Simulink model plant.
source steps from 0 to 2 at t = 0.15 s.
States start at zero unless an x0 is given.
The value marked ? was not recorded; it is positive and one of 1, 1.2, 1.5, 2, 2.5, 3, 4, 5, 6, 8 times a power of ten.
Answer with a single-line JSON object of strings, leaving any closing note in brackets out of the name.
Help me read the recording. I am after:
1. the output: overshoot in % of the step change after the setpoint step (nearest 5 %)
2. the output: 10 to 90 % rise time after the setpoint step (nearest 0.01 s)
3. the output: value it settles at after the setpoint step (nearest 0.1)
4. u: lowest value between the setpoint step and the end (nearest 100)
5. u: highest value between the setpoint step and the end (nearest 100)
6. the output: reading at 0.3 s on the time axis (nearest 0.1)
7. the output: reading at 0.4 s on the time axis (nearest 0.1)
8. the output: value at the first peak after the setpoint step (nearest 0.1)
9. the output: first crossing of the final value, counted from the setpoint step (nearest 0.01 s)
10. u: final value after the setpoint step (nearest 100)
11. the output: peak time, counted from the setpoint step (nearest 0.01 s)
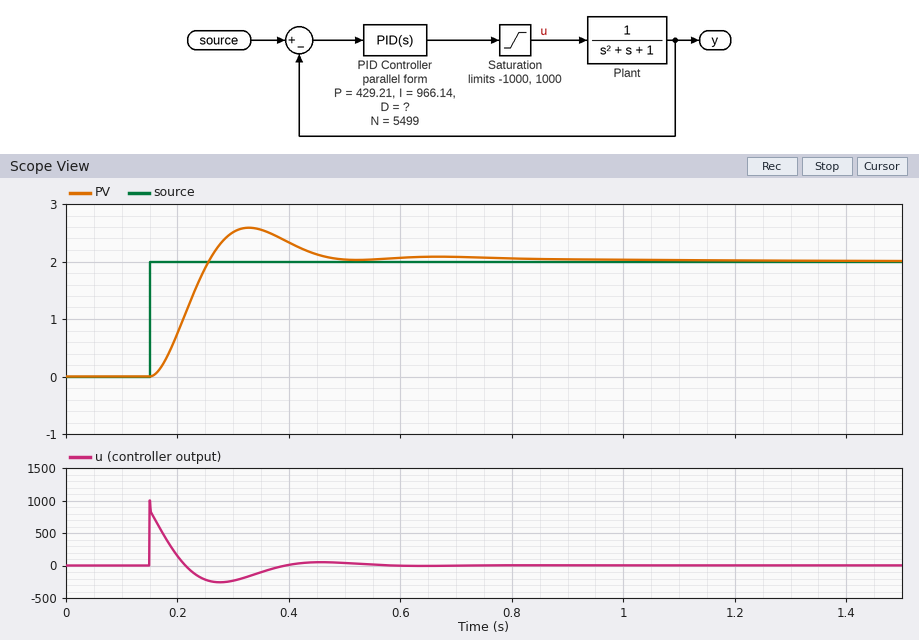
{"the output: overshoot in % of the step change after the setpoint step": "30 %", "the output: 10 to 90 % rise time after the setpoint step": "0.07 s", "the output: value it settles at after the setpoint step": "2.0", "u: lowest value between the setpoint step and the end": "-300", "u: highest value between the setpoint step and the end": "1000", "the output: reading at 0.3 s on the time axis": "2.5", "the output: reading at 0.4 s on the time axis": "2.3", "the output: value at the first peak after the setpoint step": "2.6", "the output: first crossing of the final value, counted from the setpoint step": "0.11 s", "u: final value after the setpoint step": "0", "the output: peak time, counted from the setpoint step": "0.18 s"}
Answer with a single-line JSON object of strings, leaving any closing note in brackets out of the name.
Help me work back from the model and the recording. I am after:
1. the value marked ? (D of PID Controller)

{"the value marked ?": "20"}
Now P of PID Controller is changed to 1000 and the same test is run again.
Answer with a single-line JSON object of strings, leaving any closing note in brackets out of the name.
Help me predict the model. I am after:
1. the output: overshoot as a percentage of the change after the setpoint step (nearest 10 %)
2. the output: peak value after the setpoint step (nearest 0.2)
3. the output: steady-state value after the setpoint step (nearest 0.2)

{"the output: overshoot as a percentage of the change after the setpoint step": "40 %", "the output: peak value after the setpoint step": "2.8", "the output: steady-state value after the setpoint step": "2.0"}
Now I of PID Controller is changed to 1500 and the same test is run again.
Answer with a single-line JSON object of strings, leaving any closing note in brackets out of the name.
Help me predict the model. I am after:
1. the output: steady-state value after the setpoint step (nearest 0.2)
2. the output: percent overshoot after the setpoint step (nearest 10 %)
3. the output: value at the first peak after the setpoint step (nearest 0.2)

{"the output: steady-state value after the setpoint step": "2.0", "the output: percent overshoot after the setpoint step": "40 %", "the output: value at the first peak after the setpoint step": "2.8"}
